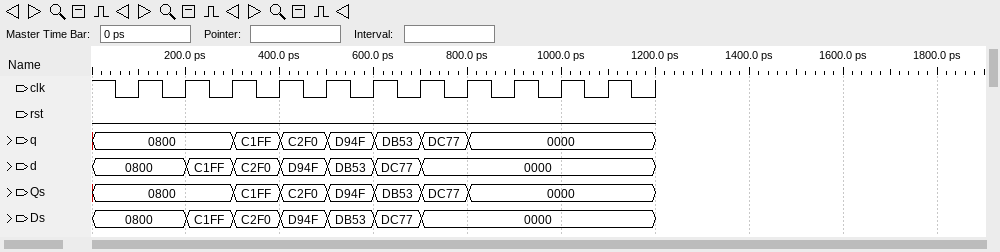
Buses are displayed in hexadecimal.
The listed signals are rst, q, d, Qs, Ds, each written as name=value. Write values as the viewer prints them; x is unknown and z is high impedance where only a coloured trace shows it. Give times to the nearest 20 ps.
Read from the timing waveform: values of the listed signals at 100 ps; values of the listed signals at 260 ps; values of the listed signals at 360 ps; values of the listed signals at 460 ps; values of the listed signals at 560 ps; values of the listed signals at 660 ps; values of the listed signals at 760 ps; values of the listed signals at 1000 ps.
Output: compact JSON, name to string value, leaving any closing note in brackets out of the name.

{"values of the listed signals at 100 ps": "rst=0, q=0800, d=0800, Qs=0800, Ds=0800", "values of the listed signals at 260 ps": "rst=0, q=0800, d=C1FF, Qs=0800, Ds=C1FF", "values of the listed signals at 360 ps": "rst=0, q=C1FF, d=C2F0, Qs=C1FF, Ds=C2F0", "values of the listed signals at 460 ps": "rst=0, q=C2F0, d=D94F, Qs=C2F0, Ds=D94F", "values of the listed signals at 560 ps": "rst=0, q=D94F, d=DB53, Qs=D94F, Ds=DB53", "values of the listed signals at 660 ps": "rst=0, q=DB53, d=DC77, Qs=DB53, Ds=DC77", "values of the listed signals at 760 ps": "rst=0, q=DC77, d=0000, Qs=DC77, Ds=0000", "values of the listed signals at 1000 ps": "rst=0, q=0000, d=0000, Qs=0000, Ds=0000"}
